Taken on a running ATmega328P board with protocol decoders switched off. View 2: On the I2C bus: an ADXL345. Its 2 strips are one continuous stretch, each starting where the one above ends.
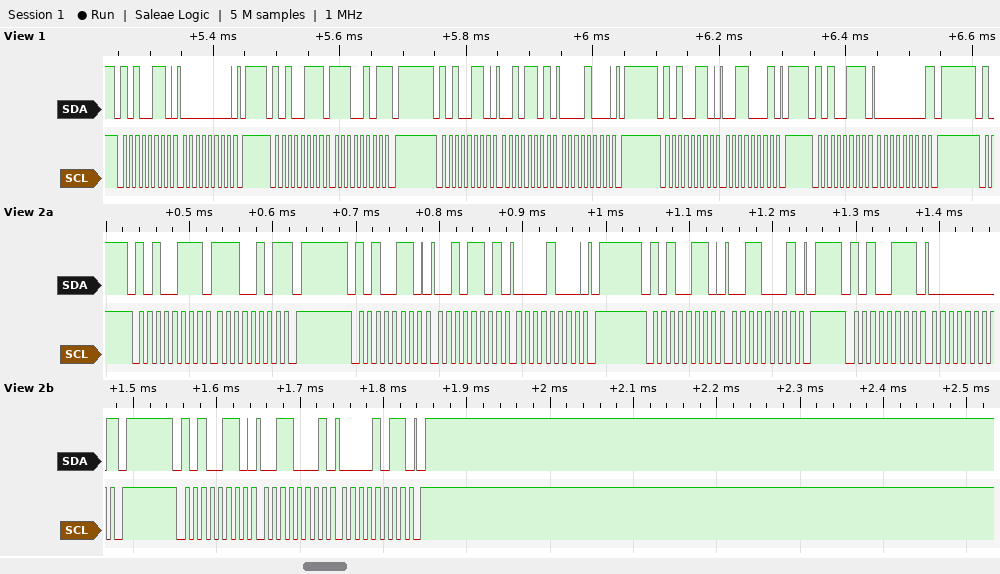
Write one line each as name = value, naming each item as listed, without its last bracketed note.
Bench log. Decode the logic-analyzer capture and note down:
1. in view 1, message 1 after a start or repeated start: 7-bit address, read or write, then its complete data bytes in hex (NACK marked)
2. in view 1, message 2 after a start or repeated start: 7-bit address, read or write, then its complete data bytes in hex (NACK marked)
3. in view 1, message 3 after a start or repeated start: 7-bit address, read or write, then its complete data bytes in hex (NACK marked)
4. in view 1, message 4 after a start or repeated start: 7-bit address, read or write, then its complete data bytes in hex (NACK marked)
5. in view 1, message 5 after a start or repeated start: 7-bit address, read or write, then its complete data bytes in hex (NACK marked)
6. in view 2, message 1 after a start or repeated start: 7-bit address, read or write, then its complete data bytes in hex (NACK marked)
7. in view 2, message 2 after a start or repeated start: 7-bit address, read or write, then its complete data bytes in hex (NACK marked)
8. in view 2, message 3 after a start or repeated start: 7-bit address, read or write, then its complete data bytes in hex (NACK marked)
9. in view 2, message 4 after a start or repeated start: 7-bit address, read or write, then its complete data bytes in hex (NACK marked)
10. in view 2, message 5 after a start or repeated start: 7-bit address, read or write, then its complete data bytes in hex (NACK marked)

in view 1, message 1 after a start or repeated start: 7-bit address, read or write, then its complete data bytes in hex = 0x53 write: 00
in view 1, message 2 after a start or repeated start: 7-bit address, read or write, then its complete data bytes in hex = 0x53 read: E5 NACK
in view 1, message 3 after a start or repeated start: 7-bit address, read or write, then its complete data bytes in hex = 0x53 write: 2D 08
in view 1, message 4 after a start or repeated start: 7-bit address, read or write, then its complete data bytes in hex = 0x53 write: 31
in view 1, message 5 after a start or repeated start: 7-bit address, read or write, then its complete data bytes in hex = 0x53 read: 00 NACK
in view 2, message 1 after a start or repeated start: 7-bit address, read or write, then its complete data bytes in hex = 0x53 read: E5 NACK
in view 2, message 2 after a start or repeated start: 7-bit address, read or write, then its complete data bytes in hex = 0x53 write: 2D 08
in view 2, message 3 after a start or repeated start: 7-bit address, read or write, then its complete data bytes in hex = 0x53 write: 31
in view 2, message 4 after a start or repeated start: 7-bit address, read or write, then its complete data bytes in hex = 0x53 read: 00 NACK
in view 2, message 5 after a start or repeated start: 7-bit address, read or write, then its complete data bytes in hex = 0x53 write: 31 0B
